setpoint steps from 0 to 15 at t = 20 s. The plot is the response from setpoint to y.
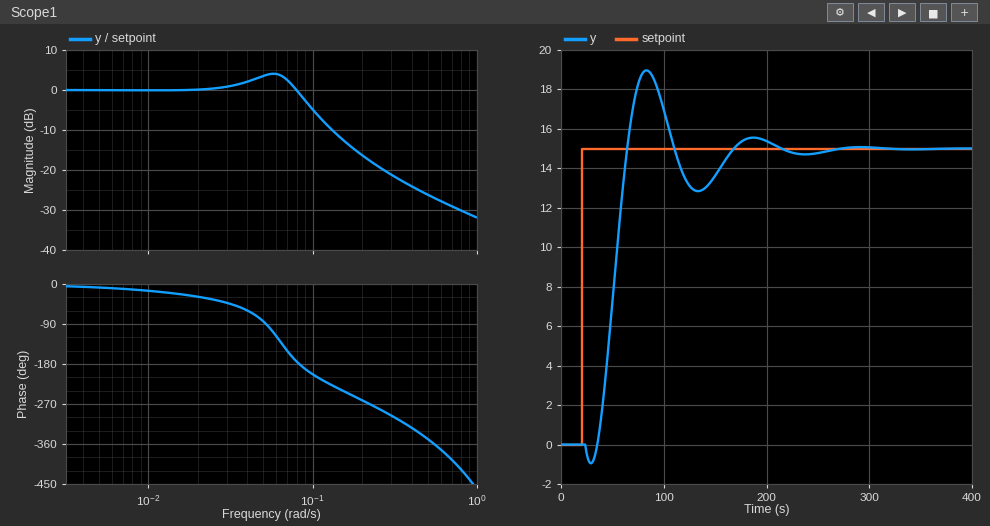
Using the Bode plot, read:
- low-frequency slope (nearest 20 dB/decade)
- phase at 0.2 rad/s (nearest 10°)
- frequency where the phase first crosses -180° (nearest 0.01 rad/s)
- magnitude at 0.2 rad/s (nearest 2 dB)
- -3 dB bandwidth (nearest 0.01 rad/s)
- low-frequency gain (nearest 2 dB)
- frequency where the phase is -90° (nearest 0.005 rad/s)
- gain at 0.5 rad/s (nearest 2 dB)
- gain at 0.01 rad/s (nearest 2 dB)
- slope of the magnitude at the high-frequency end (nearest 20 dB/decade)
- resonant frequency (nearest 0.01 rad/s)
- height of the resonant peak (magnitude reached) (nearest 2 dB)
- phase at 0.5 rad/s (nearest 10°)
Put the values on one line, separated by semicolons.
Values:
0 dB/decade; -260°; 0.08 rad/s; -16 dB; 0.09 rad/s; 0 dB; 0.050 rad/s; -26 dB; 0 dB; -20 dB/decade; 0.06 rad/s; 4 dB; -350°
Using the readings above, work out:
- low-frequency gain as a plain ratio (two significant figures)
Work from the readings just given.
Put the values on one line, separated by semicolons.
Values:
1.0
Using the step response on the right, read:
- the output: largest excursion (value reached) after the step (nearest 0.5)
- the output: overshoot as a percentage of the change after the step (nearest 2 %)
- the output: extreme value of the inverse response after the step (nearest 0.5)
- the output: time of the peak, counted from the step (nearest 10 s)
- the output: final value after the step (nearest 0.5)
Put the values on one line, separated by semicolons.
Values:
19.0; 26 %; -1.0; 60 s; 15.0
